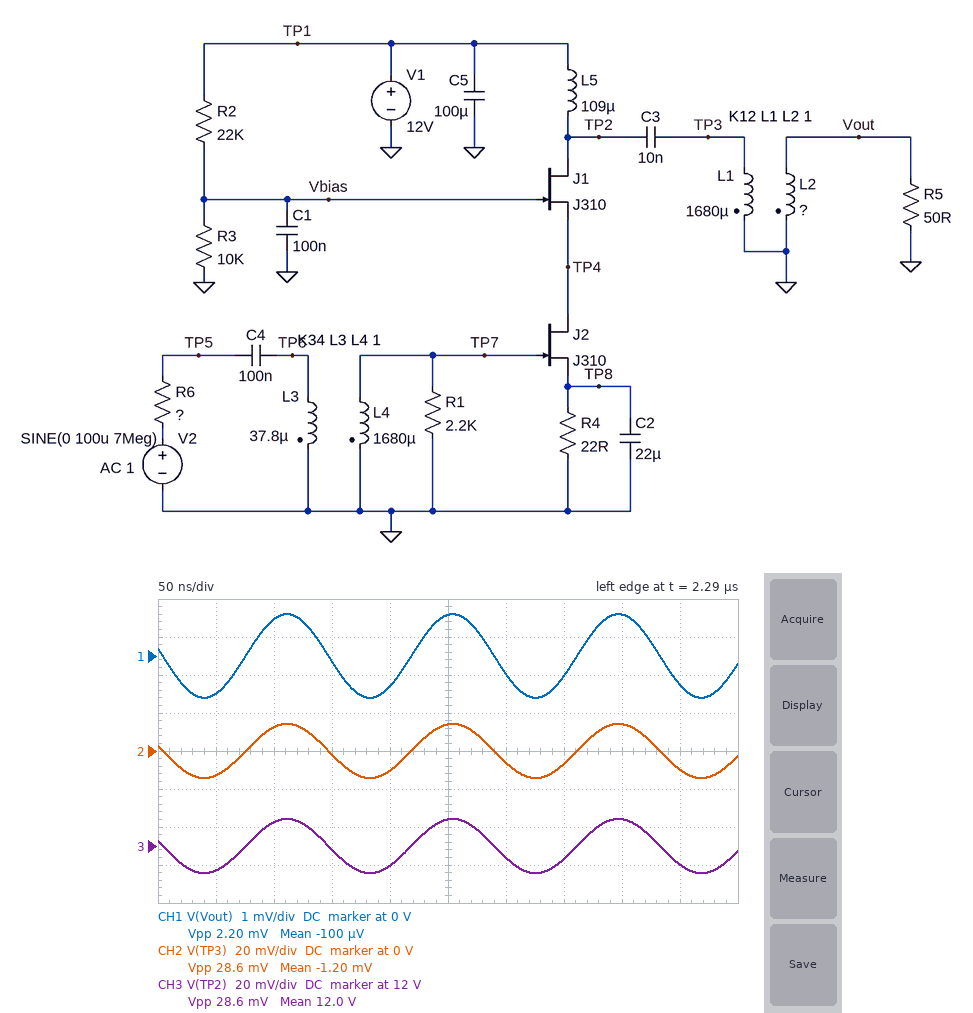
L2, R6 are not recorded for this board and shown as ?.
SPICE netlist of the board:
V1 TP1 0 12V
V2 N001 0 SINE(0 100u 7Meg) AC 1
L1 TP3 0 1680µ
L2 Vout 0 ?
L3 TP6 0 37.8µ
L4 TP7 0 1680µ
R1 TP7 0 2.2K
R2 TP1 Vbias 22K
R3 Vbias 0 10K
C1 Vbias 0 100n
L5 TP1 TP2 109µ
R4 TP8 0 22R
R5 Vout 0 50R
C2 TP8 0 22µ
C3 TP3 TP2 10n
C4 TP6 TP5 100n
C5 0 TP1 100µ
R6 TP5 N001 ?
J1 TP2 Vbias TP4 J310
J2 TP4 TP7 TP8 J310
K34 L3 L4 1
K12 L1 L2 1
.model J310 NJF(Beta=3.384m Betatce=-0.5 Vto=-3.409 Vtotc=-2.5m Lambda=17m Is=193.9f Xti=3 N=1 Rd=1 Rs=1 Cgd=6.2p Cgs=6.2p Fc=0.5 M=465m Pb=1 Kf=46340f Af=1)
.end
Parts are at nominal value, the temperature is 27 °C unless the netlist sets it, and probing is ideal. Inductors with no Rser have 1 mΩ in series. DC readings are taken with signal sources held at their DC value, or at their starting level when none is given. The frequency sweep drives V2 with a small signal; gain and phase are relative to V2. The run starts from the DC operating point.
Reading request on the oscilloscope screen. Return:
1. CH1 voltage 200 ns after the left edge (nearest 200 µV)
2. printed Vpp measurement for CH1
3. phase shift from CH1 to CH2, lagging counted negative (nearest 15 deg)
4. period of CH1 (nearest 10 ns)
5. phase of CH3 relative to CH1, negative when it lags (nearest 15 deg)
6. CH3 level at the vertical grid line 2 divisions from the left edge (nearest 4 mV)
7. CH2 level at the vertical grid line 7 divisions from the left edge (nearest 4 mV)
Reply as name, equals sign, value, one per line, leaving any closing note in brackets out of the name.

CH1 voltage 200 ns after the left edge = -800 µV
printed Vpp measurement for CH1 = 2.20 mV
phase shift from CH1 to CH2, lagging counted negative = 0 deg
period of CH1 = 140 ns
phase of CH3 relative to CH1, negative when it lags = 0 deg
CH3 level at the vertical grid line 2 divisions from the left edge = 12.012 V
CH2 level at the vertical grid line 7 divisions from the left edge = -8 mV
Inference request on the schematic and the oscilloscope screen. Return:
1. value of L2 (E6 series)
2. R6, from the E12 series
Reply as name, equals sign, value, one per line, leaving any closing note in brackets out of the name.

value of L2 = 10 µH
R6, from the E12 series = 150 Ω
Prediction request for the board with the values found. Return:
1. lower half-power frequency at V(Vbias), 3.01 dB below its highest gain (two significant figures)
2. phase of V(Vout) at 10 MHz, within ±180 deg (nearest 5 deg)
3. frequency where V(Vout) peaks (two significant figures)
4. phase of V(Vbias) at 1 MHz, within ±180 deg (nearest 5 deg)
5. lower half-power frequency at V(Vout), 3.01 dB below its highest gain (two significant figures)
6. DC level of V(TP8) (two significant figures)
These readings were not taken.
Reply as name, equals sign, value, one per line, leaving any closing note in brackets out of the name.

lower half-power frequency at V(Vbias), 3.01 dB below its highest gain = 4.5 MHz
phase of V(Vout) at 10 MHz, within ±180 deg = 125 deg
frequency where V(Vout) peaks = 7.4 MHz
phase of V(Vbias) at 1 MHz, within ±180 deg = -100 deg
lower half-power frequency at V(Vout), 3.01 dB below its highest gain = 4.5 MHz
DC level of V(TP8) = 610 mV
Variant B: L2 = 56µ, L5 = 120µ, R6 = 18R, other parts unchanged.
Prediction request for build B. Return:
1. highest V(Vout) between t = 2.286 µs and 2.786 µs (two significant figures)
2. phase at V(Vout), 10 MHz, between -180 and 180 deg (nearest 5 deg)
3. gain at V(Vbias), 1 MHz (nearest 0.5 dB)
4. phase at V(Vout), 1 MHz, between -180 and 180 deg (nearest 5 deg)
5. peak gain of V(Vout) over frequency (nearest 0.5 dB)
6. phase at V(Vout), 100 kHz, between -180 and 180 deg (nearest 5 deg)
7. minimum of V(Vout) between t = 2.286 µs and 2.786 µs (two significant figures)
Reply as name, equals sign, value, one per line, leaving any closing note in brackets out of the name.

highest V(Vout) between t = 2.286 µs and 2.786 µs = 2.4 mV
phase at V(Vout), 10 MHz, between -180 and 180 deg = 155 deg
gain at V(Vbias), 1 MHz = -57.0 dB
phase at V(Vout), 1 MHz, between -180 and 180 deg = -115 deg
peak gain of V(Vout) over frequency = 27.5 dB
phase at V(Vout), 100 kHz, between -180 and 180 deg = -30 deg
minimum of V(Vout) between t = 2.286 µs and 2.786 µs = -2.4 mV
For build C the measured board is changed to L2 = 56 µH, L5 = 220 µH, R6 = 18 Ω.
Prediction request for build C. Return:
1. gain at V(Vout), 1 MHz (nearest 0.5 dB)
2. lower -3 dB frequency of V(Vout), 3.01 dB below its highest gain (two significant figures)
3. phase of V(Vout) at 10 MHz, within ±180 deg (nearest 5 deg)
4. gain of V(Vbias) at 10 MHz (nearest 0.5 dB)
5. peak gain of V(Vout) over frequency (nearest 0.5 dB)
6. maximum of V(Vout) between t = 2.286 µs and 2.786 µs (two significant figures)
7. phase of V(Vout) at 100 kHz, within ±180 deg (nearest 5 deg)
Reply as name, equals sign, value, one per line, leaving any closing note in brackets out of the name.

gain at V(Vout), 1 MHz = 24.5 dB
lower -3 dB frequency of V(Vout), 3.01 dB below its highest gain = 1.1 MHz
phase of V(Vout) at 10 MHz, within ±180 deg = 150 deg
gain of V(Vbias) at 10 MHz = -51.0 dB
peak gain of V(Vout) over frequency = 28.0 dB
maximum of V(Vout) between t = 2.286 µs and 2.786 µs = 2.4 mV
phase of V(Vout) at 100 kHz, within ±180 deg = -30 deg
